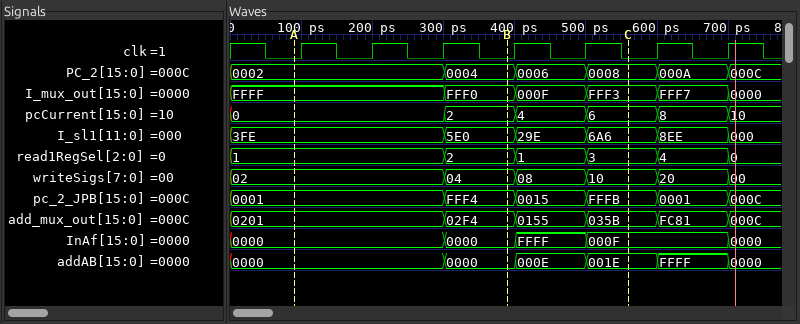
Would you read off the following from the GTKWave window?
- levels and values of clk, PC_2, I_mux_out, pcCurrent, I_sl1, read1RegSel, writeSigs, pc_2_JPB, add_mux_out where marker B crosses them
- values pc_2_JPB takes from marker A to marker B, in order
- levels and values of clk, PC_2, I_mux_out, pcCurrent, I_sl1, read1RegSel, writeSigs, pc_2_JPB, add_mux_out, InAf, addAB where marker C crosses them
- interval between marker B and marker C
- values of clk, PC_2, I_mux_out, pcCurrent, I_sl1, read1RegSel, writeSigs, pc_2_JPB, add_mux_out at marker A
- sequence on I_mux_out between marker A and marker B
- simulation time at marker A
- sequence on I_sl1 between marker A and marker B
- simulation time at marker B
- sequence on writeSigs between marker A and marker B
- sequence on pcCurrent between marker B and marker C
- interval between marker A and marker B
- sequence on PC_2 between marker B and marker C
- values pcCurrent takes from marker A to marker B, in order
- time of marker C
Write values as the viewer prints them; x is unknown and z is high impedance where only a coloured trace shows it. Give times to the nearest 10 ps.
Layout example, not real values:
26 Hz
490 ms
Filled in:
clk=0, PC_2=0004, I_mux_out=FFF0, pcCurrent=2, I_sl1=5E0, read1RegSel=2, writeSigs=04, pc_2_JPB=FFF4, add_mux_out=02F4
0001, FFF4
clk=0, PC_2=0008, I_mux_out=FFF3, pcCurrent=6, I_sl1=6A6, read1RegSel=3, writeSigs=10, pc_2_JPB=FFFB, add_mux_out=035B, InAf=000F, addAB=001E
170 ps
clk=0, PC_2=0002, I_mux_out=FFFF, pcCurrent=0, I_sl1=3FE, read1RegSel=1, writeSigs=02, pc_2_JPB=0001, add_mux_out=0201
FFFF, FFF0
90 ps
3FE, 5E0
390 ps
02, 04
2, 4, 6
300 ps
0004, 0006, 0008
0, 2
560 ps
